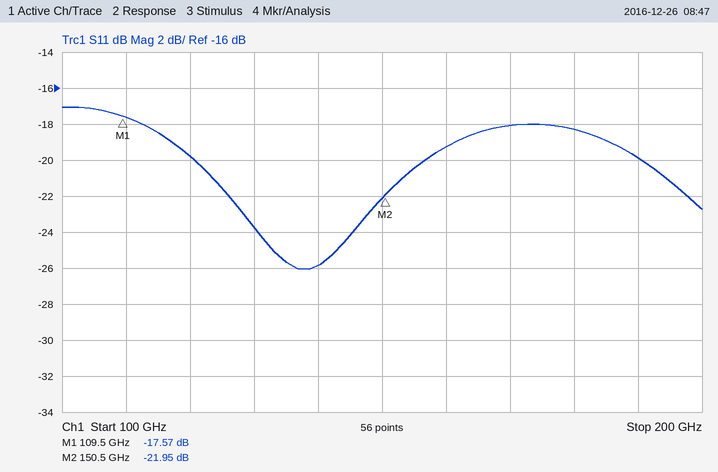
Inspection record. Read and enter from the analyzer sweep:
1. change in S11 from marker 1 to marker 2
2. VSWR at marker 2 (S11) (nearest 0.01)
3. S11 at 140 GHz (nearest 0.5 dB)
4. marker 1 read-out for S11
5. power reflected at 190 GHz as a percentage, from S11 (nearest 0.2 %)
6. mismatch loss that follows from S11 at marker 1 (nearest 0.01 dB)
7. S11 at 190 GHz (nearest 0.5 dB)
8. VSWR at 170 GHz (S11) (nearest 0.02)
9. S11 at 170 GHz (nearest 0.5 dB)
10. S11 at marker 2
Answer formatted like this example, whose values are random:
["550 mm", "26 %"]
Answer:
["-4.38 dB", "1.17", "-26.0 dB", "-17.57 dB", "1.0 %", "0.08 dB", "-20.0 dB", "1.28", "-18.0 dB", "-21.95 dB"]
